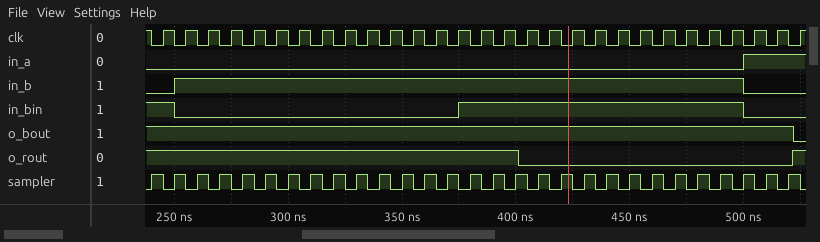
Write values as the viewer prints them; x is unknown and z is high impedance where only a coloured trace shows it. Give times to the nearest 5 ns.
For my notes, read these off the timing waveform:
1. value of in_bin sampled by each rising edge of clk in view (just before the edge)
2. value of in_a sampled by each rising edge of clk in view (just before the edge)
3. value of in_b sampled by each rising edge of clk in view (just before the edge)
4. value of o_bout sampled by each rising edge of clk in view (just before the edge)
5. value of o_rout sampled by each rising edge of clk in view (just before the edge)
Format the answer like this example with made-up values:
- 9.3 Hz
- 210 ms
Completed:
- 1 0 0 0 0 0 0 0 0 0 0 0 0 0 1 1 1 1 1 1 1 1 1 1 1 1 0 0 0
- 0 0 0 0 0 0 0 0 0 0 0 0 0 0 0 0 0 0 0 0 0 0 0 0 0 0 1 1 1
- 0 1 1 1 1 1 1 1 1 1 1 1 1 1 1 1 1 1 1 1 1 1 1 1 1 1 0 0 0
- 1 1 1 1 1 1 1 1 1 1 1 1 1 1 1 1 1 1 1 1 1 1 1 1 1 1 1 1 0
- 1 1 1 1 1 1 1 1 1 1 1 1 1 1 1 1 0 0 0 0 0 0 0 0 0 0 0 0 1
